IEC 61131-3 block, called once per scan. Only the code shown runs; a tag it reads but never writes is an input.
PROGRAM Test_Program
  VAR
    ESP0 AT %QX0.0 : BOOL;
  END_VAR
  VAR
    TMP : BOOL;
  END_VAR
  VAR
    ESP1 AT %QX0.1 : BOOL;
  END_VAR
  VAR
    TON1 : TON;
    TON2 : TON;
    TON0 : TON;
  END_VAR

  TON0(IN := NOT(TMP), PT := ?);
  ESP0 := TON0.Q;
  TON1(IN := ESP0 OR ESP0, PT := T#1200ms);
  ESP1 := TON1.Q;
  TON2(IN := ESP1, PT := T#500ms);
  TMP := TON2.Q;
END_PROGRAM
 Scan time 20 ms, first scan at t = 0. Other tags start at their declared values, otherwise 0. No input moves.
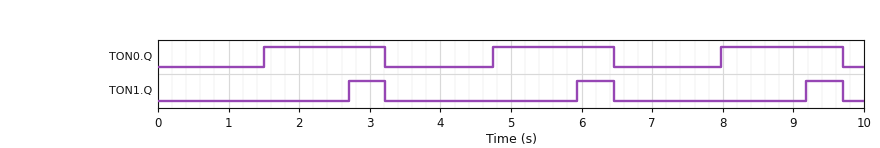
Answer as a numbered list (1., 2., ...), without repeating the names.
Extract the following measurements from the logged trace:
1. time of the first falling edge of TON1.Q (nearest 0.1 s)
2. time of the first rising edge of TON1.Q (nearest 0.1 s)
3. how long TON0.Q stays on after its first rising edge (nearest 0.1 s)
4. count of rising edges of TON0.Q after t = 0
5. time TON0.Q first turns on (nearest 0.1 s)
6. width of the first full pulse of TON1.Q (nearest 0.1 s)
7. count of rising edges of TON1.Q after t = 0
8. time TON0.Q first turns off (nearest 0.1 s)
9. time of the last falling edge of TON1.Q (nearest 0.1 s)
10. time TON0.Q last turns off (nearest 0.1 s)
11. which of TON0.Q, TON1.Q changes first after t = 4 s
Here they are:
1. 3.2 s
2. 2.7 s
3. 1.7 s
4. 3
5. 1.5 s
6. 0.5 s
7. 3
8. 3.2 s
9. 9.7 s
10. 9.7 s
11. TON0.Q
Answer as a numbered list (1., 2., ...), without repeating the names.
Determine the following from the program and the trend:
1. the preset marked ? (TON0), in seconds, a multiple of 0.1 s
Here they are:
1. 1.5 s
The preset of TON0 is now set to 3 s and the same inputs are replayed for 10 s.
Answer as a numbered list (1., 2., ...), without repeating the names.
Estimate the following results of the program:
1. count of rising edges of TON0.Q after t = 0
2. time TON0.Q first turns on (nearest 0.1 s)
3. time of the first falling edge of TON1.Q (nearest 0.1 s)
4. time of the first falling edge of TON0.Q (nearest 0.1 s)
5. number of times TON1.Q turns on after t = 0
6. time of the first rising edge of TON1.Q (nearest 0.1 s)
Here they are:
1. 2
2. 3.0 s
3. 4.7 s
4. 4.7 s
5. 2
6. 4.2 s
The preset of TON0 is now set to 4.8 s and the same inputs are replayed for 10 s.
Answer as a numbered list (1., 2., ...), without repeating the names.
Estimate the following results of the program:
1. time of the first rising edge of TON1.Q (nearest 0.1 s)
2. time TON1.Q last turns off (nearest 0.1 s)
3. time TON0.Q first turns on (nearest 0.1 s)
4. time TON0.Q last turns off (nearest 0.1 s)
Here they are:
1. 6.0 s
2. 6.5 s
3. 4.8 s
4. 6.5 s
